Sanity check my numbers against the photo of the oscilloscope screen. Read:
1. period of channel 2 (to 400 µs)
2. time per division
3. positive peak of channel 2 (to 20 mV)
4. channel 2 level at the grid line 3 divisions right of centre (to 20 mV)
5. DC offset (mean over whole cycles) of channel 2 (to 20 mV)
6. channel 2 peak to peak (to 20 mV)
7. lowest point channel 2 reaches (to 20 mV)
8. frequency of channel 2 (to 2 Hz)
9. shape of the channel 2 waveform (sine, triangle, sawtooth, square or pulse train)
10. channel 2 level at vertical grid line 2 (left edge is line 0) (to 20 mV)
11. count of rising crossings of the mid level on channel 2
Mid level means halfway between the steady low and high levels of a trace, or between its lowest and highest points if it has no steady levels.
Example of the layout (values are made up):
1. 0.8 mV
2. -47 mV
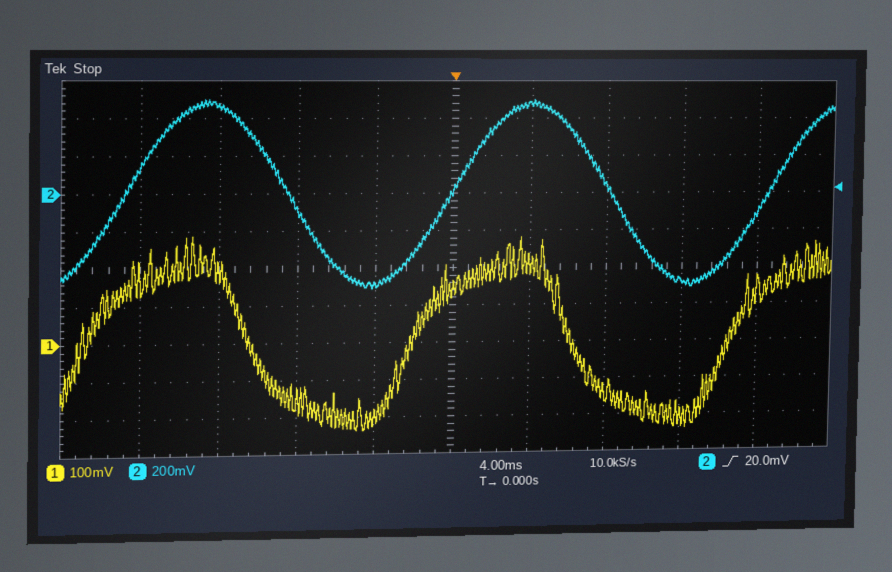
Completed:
1. 16.8 ms
2. 4 ms
3. 500 mV
4. -480 mV
5. 0 mV
6. 1.00 V
7. -500 mV
8. 60 Hz
9. sine
10. 460 mV
11. 3
